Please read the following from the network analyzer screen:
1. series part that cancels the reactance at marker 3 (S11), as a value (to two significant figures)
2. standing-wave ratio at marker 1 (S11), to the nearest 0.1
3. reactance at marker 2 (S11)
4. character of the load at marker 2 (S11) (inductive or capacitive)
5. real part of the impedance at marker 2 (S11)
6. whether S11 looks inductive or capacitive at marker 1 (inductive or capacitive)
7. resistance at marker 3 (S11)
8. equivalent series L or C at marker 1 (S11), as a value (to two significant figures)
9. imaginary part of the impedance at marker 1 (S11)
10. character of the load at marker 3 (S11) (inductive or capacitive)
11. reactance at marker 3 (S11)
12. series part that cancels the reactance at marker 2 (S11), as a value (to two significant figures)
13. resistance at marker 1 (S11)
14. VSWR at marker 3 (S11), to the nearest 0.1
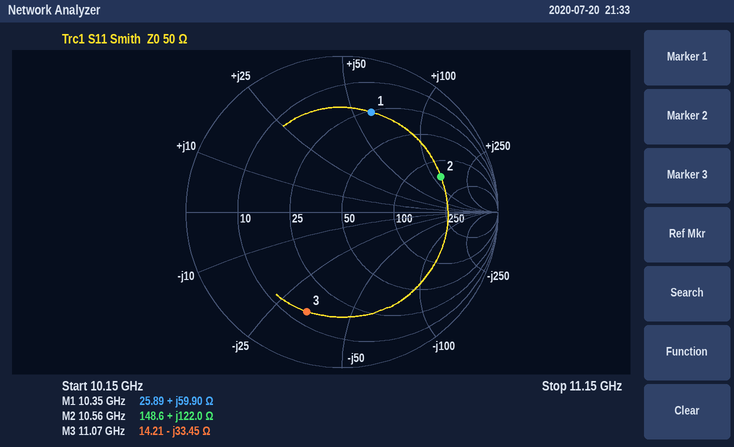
480 pH
5.0
+122.0 Ω
inductive
148.6 Ω
inductive
14.21 Ω
920 pH
+59.90 Ω
capacitive
-33.45 Ω
120 fF
25.89 Ω
5.2
